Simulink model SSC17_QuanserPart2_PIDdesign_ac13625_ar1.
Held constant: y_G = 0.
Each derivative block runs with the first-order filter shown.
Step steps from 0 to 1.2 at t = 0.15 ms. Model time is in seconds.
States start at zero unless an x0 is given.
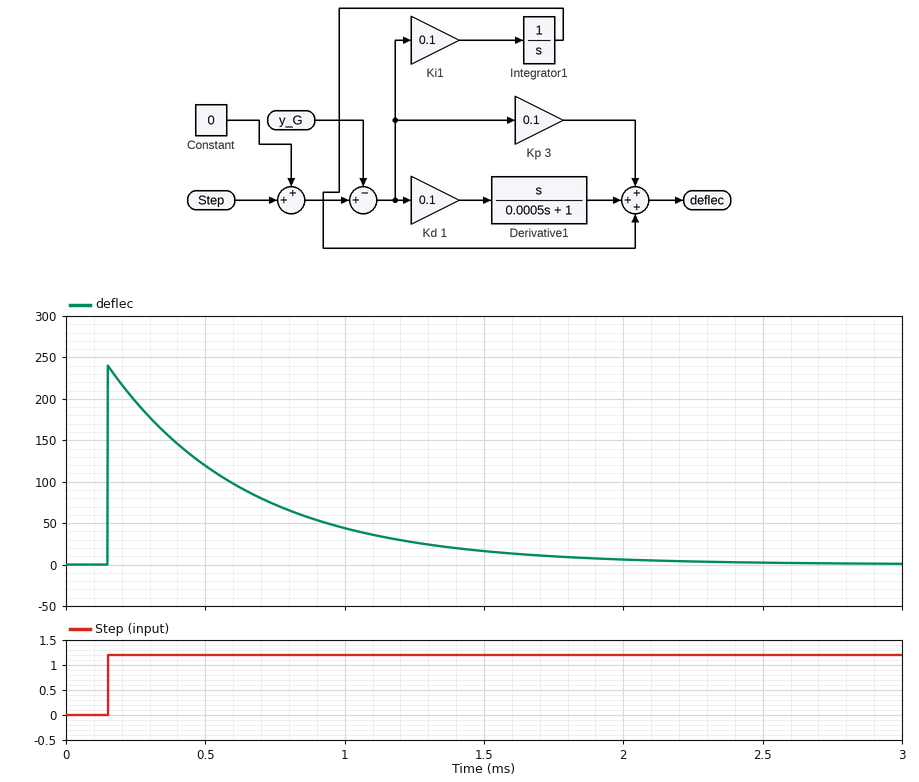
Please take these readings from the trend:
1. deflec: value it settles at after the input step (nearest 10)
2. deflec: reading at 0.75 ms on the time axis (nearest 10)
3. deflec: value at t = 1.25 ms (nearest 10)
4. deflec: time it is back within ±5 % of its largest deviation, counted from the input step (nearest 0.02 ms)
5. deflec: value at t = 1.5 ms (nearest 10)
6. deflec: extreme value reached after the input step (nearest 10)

0
70
30
1.50 ms
20
240
